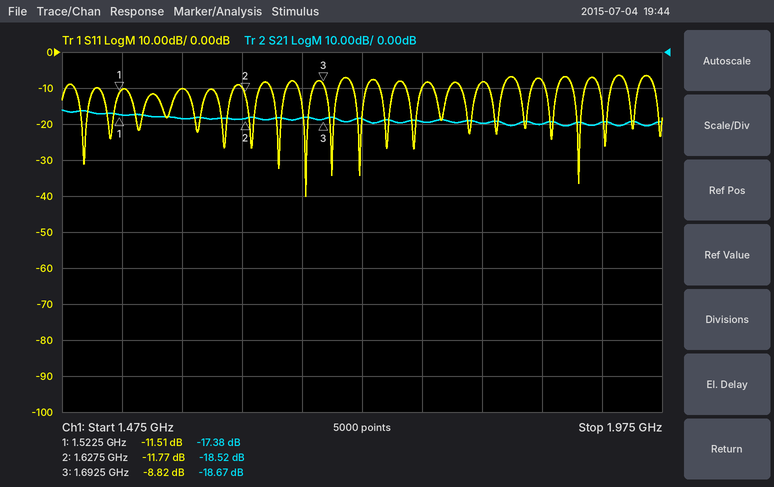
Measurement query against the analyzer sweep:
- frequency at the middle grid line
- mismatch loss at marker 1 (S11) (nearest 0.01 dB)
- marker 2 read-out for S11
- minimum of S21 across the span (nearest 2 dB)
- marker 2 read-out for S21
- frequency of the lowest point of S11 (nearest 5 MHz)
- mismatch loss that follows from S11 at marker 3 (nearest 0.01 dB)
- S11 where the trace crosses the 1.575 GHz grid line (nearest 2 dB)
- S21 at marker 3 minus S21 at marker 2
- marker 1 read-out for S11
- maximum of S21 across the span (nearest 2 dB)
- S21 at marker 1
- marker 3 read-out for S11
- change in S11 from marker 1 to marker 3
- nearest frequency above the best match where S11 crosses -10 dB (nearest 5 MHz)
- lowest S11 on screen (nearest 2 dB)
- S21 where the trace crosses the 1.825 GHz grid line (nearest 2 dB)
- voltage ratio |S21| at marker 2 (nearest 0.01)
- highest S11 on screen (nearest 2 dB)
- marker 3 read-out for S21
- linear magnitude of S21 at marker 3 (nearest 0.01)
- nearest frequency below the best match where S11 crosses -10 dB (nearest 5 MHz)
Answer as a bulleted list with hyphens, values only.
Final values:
- 1.725 GHz
- 0.32 dB
- -11.77 dB
- -20 dB
- -18.52 dB
- 1.680 GHz
- 0.61 dB
- -10 dB
- -0.15 dB
- -11.51 dB
- -16 dB
- -17.38 dB
- -8.82 dB
- 2.69 dB
- 1.685 GHz
- -40 dB
- -20 dB
- 0.12
- -6 dB
- -18.67 dB
- 0.12
- 1.670 GHz
